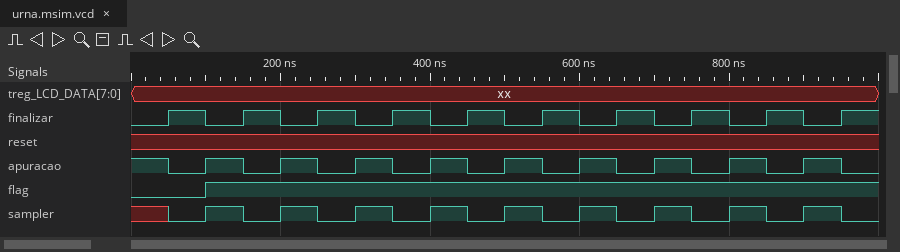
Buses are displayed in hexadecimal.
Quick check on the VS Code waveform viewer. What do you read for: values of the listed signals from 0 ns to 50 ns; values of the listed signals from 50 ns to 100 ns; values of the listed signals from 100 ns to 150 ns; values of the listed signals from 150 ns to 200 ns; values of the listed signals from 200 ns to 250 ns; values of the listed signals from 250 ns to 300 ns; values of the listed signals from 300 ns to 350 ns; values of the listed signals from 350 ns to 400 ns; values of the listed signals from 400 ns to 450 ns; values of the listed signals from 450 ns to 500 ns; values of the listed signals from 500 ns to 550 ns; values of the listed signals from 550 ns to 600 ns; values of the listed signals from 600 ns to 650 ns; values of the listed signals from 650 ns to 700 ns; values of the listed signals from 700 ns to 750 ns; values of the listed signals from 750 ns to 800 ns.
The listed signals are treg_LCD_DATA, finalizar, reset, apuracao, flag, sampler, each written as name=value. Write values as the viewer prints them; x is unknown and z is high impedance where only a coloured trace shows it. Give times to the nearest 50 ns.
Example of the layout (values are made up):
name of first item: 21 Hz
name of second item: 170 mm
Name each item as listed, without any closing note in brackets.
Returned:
values of the listed signals from 0 ns to 50 ns: treg_LCD_DATA=xx, finalizar=0, reset=x, apuracao=1, flag=0, sampler=x
values of the listed signals from 50 ns to 100 ns: treg_LCD_DATA=xx, finalizar=1, reset=x, apuracao=0, flag=0, sampler=0
values of the listed signals from 100 ns to 150 ns: treg_LCD_DATA=xx, finalizar=0, reset=x, apuracao=1, flag=1, sampler=1
values of the listed signals from 150 ns to 200 ns: treg_LCD_DATA=xx, finalizar=1, reset=x, apuracao=0, flag=1, sampler=0
values of the listed signals from 200 ns to 250 ns: treg_LCD_DATA=xx, finalizar=0, reset=x, apuracao=1, flag=1, sampler=1
values of the listed signals from 250 ns to 300 ns: treg_LCD_DATA=xx, finalizar=1, reset=x, apuracao=0, flag=1, sampler=0
values of the listed signals from 300 ns to 350 ns: treg_LCD_DATA=xx, finalizar=0, reset=x, apuracao=1, flag=1, sampler=1
values of the listed signals from 350 ns to 400 ns: treg_LCD_DATA=xx, finalizar=1, reset=x, apuracao=0, flag=1, sampler=0
values of the listed signals from 400 ns to 450 ns: treg_LCD_DATA=xx, finalizar=0, reset=x, apuracao=1, flag=1, sampler=1
values of the listed signals from 450 ns to 500 ns: treg_LCD_DATA=xx, finalizar=1, reset=x, apuracao=0, flag=1, sampler=0
values of the listed signals from 500 ns to 550 ns: treg_LCD_DATA=xx, finalizar=0, reset=x, apuracao=1, flag=1, sampler=1
values of the listed signals from 550 ns to 600 ns: treg_LCD_DATA=xx, finalizar=1, reset=x, apuracao=0, flag=1, sampler=0
values of the listed signals from 600 ns to 650 ns: treg_LCD_DATA=xx, finalizar=0, reset=x, apuracao=1, flag=1, sampler=1
values of the listed signals from 650 ns to 700 ns: treg_LCD_DATA=xx, finalizar=1, reset=x, apuracao=0, flag=1, sampler=0
values of the listed signals from 700 ns to 750 ns: treg_LCD_DATA=xx, finalizar=0, reset=x, apuracao=1, flag=1, sampler=1
values of the listed signals from 750 ns to 800 ns: treg_LCD_DATA=xx, finalizar=1, reset=x, apuracao=0, flag=1, sampler=0
